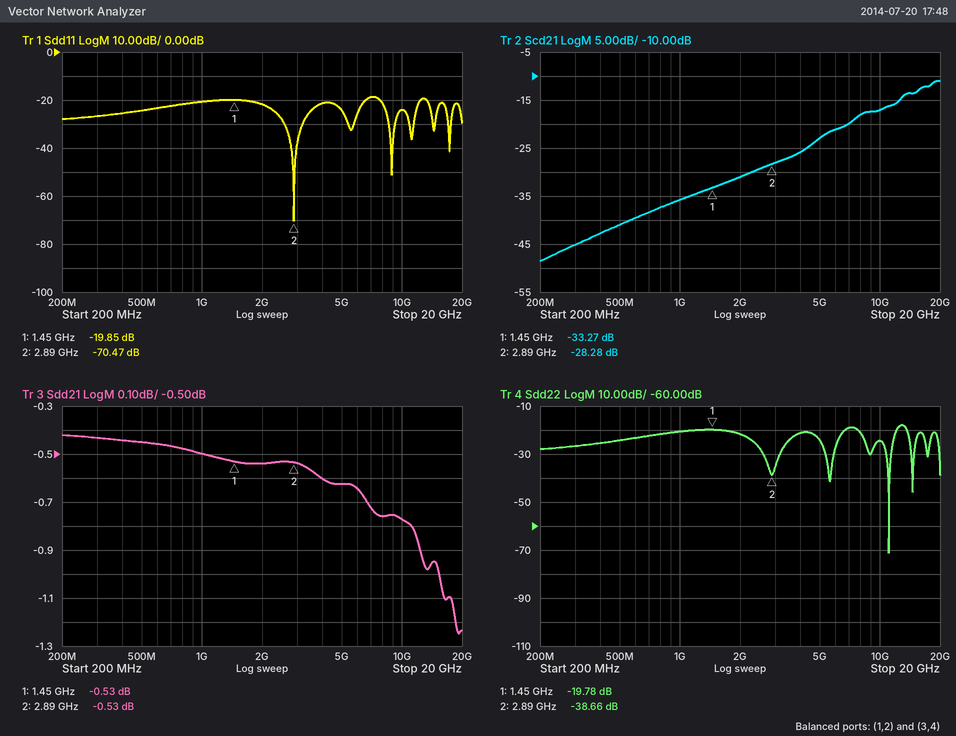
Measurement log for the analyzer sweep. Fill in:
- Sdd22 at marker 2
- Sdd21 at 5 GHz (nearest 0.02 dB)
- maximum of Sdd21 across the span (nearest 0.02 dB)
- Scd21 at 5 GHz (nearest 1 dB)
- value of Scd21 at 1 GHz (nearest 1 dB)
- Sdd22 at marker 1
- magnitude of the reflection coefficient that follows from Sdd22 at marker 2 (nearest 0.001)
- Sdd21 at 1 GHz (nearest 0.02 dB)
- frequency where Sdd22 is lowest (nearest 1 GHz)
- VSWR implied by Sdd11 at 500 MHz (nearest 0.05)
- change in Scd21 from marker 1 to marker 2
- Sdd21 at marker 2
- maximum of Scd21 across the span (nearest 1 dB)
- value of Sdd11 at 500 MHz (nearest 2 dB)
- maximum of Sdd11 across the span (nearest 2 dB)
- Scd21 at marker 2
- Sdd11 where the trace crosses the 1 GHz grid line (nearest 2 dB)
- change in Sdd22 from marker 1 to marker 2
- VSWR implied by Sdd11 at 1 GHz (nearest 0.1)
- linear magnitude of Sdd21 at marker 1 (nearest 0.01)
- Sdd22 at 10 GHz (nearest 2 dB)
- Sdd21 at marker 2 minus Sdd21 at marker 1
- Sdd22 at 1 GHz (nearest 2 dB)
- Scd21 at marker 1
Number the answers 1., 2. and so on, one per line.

1. -38.66 dB
2. -0.62 dB
3. -0.42 dB
4. -23 dB
5. -36 dB
6. -19.78 dB
7. 0.012
8. -0.50 dB
9. 11 GHz
10. 1.15
11. 4.99 dB
12. -0.53 dB
13. -11 dB
14. -24 dB
15. -18 dB
16. -28.28 dB
17. -20 dB
18. -18.88 dB
19. 1.2
20. 0.94
21. -24 dB
22. 0.00 dB
23. -20 dB
24. -33.27 dB
